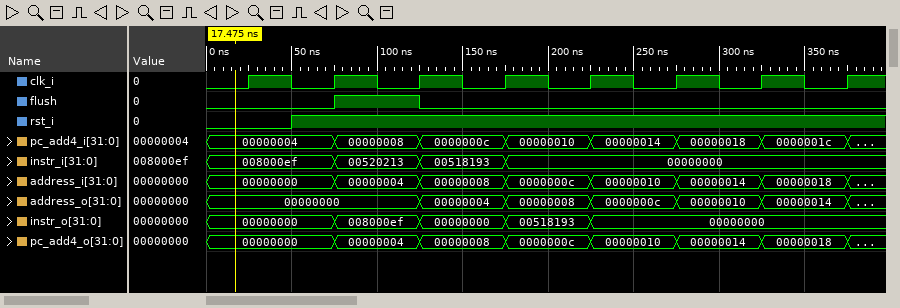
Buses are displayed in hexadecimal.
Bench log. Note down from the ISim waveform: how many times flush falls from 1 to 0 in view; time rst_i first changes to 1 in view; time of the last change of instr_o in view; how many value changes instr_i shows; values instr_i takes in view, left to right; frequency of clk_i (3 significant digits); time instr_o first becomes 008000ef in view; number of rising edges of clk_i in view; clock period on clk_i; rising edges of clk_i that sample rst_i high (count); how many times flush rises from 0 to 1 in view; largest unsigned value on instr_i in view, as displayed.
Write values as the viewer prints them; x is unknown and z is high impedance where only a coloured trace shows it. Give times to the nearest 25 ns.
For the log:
1
50 ns
225 ns
3
008000ef, 00520213, 00518193, 00000000
20.0 MHz
75 ns
8
50 ns
7
1
008000ef
